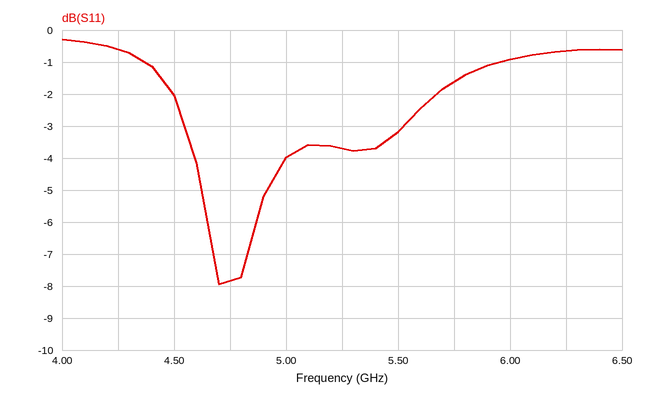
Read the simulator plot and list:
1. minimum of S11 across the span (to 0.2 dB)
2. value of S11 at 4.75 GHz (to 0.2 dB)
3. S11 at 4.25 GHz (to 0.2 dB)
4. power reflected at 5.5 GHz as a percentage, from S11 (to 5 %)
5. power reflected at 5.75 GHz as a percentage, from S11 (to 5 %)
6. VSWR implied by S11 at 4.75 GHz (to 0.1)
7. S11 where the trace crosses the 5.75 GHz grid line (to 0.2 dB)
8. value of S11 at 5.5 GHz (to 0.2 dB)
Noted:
-8.0 dB
-7.8 dB
-0.6 dB
50 %
70 %
2.4
-1.6 dB
-3.2 dB
